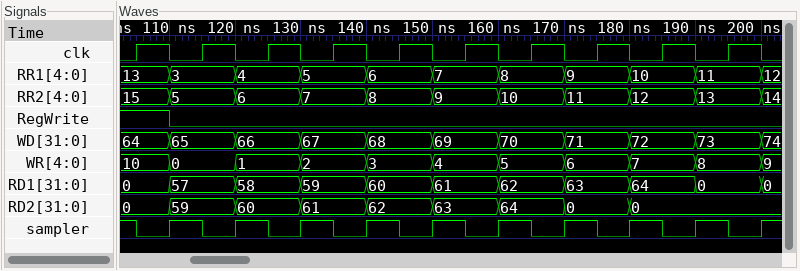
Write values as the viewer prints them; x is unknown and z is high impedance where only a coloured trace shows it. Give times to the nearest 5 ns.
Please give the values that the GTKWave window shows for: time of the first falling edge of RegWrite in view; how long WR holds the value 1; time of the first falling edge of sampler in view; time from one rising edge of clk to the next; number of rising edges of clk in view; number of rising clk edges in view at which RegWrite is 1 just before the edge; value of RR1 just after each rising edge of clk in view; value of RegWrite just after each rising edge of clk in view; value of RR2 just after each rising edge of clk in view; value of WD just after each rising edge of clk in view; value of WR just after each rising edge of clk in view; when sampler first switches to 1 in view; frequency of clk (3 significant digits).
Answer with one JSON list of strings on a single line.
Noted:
["110 ns", "10 ns", "105 ns", "10 ns", "10", "1", "13, 3, 4, 5, 6, 7, 8, 9, 10, 11", "1 0 0 0 0 0 0 0 0 0", "15, 5, 6, 7, 8, 9, 10, 11, 12, 13", "64, 65, 66, 67, 68, 69, 70, 71, 72, 73", "10, 0, 1, 2, 3, 4, 5, 6, 7, 8", "110 ns", "100 MHz"]
